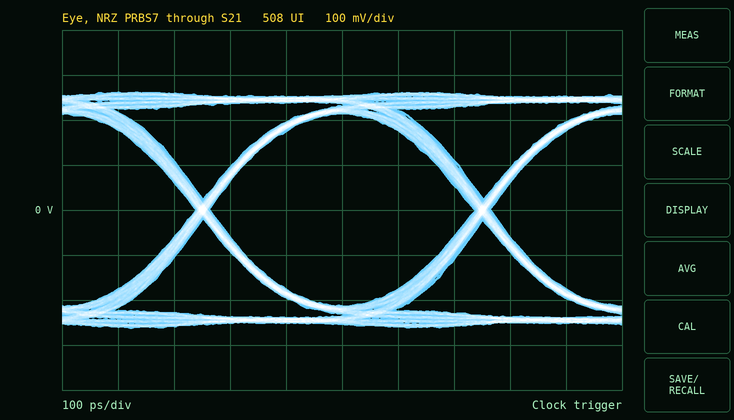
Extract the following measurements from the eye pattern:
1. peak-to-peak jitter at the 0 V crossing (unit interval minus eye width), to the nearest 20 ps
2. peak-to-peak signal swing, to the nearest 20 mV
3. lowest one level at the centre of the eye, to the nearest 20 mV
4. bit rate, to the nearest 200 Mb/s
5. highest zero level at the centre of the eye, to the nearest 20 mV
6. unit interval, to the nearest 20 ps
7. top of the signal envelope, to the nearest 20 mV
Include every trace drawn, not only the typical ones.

20 ps
520 mV
220 mV
2.0 Gb/s
-220 mV
500 ps
260 mV
